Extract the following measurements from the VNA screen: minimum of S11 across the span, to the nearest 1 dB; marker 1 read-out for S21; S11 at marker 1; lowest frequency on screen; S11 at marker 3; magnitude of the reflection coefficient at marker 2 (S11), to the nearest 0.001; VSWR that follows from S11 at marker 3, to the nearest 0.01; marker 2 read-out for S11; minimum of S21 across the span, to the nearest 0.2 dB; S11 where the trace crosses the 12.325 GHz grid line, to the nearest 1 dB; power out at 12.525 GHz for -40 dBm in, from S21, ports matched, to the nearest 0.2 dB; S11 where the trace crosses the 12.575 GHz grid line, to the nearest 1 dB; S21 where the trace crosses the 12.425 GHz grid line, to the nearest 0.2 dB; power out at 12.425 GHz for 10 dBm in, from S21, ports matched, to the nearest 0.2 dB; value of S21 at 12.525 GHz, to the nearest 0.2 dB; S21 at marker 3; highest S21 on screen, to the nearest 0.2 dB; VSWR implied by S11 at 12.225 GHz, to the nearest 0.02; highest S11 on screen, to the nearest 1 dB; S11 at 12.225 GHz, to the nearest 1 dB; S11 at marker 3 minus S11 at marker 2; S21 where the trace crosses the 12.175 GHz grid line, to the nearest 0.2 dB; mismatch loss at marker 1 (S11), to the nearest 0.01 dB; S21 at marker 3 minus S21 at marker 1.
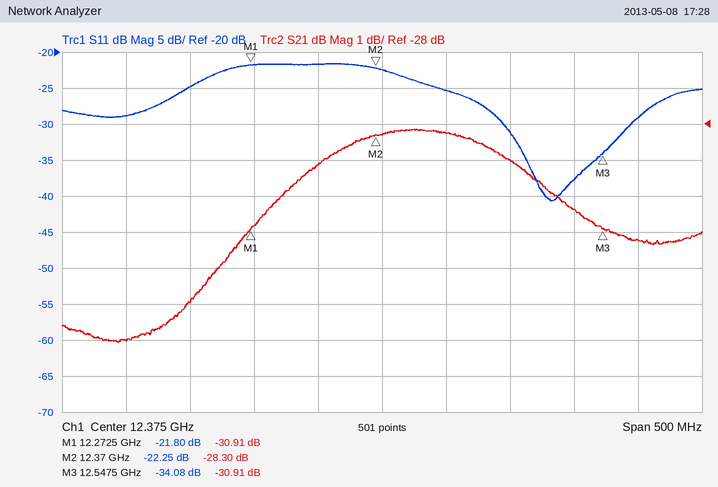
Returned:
-41 dB
-30.91 dB
-21.80 dB
12.125 GHz
-34.08 dB
0.077
1.04
-22.25 dB
-34.0 dB
-22 dB
-70.4 dBm
-29 dB
-28.2 dB
-18.2 dBm
-30.4 dB
-30.91 dB
-28.2 dB
1.12
-22 dB
-25 dB
-11.83 dB
-34.0 dB
0.03 dB
0.00 dB
